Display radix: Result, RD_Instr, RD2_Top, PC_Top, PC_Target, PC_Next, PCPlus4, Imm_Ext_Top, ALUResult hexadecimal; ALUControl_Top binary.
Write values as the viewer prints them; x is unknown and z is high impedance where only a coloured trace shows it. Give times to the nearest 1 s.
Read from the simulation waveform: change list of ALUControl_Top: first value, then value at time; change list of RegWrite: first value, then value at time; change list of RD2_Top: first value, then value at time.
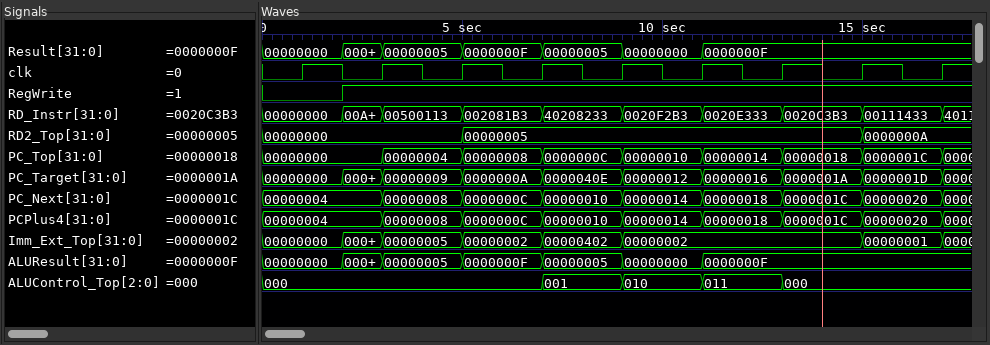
000, 001 at 7 s, 010 at 9 s, 011 at 11 s, 000 at 13 s
0, 1 at 2 s
00000000, 00000005 at 5 s, 0000000A at 15 s
